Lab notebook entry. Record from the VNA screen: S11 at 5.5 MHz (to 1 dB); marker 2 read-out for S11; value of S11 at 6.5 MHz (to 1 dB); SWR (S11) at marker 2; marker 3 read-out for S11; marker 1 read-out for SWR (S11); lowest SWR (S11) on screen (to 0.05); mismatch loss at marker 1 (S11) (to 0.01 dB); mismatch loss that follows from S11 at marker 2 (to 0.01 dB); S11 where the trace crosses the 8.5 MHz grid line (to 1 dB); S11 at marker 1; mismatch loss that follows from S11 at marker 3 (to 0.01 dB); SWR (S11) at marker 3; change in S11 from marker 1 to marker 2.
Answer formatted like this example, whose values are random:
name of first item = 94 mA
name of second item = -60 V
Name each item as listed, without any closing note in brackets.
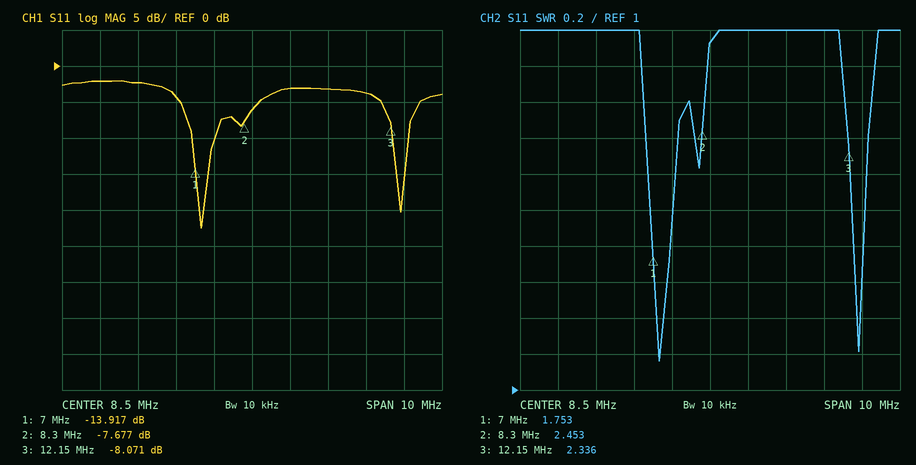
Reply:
S11 at 5.5 MHz = -2 dB
marker 2 read-out for S11 = -7.677 dB
value of S11 at 6.5 MHz = -4 dB
SWR (S11) at marker 2 = 2.453
marker 3 read-out for S11 = -8.071 dB
marker 1 read-out for SWR = 1.753
lowest SWR (S11) on screen = 1.15
mismatch loss at marker 1 (S11) = 0.18 dB
mismatch loss that follows from S11 at marker 2 = 0.81 dB
S11 where the trace crosses the 8.5 MHz grid line = -6 dB
S11 at marker 1 = -13.917 dB
mismatch loss that follows from S11 at marker 3 = 0.74 dB
SWR (S11) at marker 3 = 2.336
change in S11 from marker 1 to marker 2 = 6.240 dB
